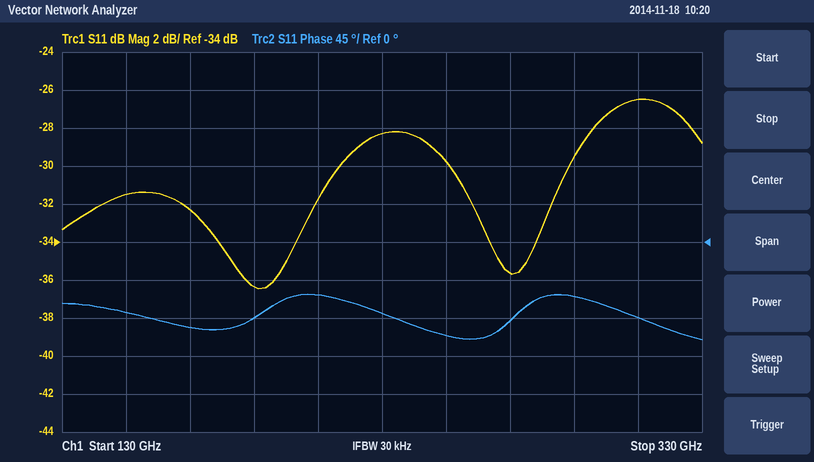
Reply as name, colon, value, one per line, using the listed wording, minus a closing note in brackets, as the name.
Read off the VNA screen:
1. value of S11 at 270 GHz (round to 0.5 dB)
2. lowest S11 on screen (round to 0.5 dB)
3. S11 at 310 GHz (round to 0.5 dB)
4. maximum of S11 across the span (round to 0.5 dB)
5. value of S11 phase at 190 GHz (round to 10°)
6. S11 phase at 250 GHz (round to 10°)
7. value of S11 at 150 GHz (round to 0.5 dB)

value of S11 at 270 GHz: -35.5 dB
lowest S11 on screen: -36.5 dB
S11 at 310 GHz: -26.5 dB
maximum of S11 across the span: -26.5 dB
value of S11 phase at 190 GHz: -90°
S11 phase at 250 GHz: -110°
value of S11 at 150 GHz: -31.5 dB
